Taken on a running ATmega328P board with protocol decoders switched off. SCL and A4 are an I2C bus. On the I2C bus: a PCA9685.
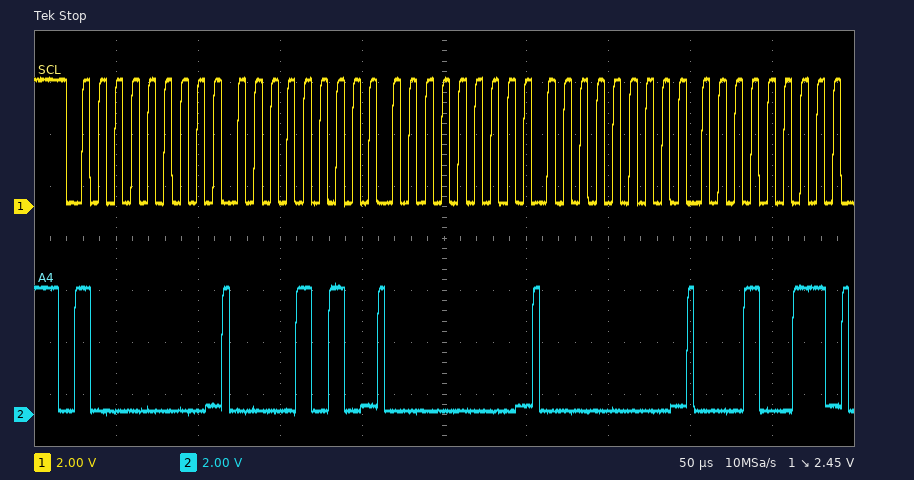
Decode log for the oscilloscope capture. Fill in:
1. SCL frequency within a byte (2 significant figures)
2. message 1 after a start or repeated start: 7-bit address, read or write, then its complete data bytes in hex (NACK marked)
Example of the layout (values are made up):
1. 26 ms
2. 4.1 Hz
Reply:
1. 100 kHz
2. 0x40 write: 0A 00 00 13
